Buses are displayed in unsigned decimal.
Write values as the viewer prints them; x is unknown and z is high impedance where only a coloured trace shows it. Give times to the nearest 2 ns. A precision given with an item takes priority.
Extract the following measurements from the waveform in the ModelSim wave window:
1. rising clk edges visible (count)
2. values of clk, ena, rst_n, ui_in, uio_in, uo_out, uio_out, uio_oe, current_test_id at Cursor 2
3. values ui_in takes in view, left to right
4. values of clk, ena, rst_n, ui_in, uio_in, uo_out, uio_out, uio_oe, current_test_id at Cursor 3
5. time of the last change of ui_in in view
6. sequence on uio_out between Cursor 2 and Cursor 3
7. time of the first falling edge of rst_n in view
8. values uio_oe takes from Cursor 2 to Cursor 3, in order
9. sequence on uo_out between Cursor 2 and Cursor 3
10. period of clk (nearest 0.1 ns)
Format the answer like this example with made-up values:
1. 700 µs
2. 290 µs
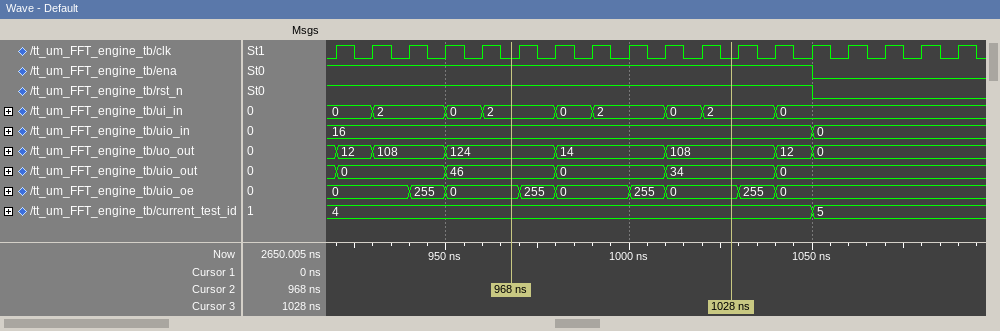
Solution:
1. 18
2. clk=0, ena=1, rst_n=1, ui_in=2, uio_in=16, uo_out=124, uio_out=46, uio_oe=0, current_test_id=4
3. 0, 2, 0, 2, 0, 2, 0, 2, 0
4. clk=0, ena=1, rst_n=1, ui_in=2, uio_in=16, uo_out=108, uio_out=34, uio_oe=0, current_test_id=4
5. 1040 ns
6. 46, 0, 34
7. 1050 ns
8. 0, 255, 0, 255, 0
9. 124, 14, 108
10. 10 ns
